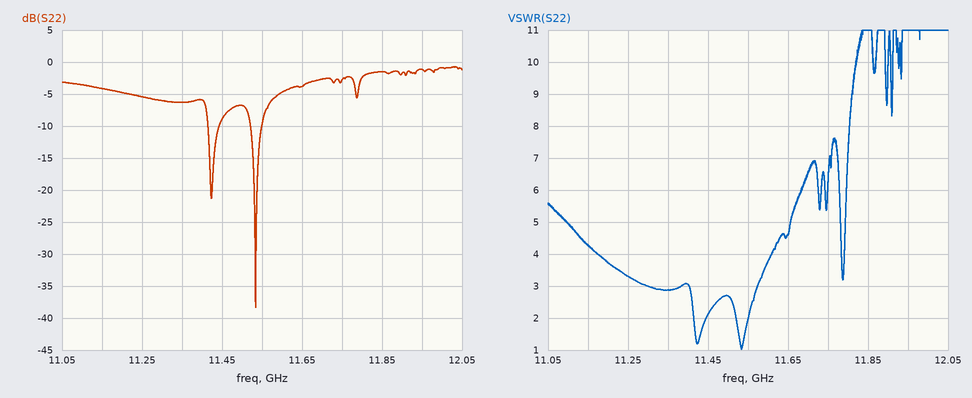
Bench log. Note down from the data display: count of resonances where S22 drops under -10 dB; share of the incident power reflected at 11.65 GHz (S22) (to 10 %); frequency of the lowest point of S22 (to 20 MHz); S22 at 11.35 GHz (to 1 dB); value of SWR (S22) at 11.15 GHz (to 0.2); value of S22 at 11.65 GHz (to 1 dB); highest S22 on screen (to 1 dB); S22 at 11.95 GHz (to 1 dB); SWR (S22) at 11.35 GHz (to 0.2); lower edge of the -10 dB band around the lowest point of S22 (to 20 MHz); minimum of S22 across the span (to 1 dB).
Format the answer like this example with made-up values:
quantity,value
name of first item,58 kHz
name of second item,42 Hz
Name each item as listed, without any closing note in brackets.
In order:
quantity,value
count of resonances where S22 drops under -10 dB,2
share of the incident power reflected at 11.65 GHz (S22),40 %
frequency of the lowest point of S22,11.54 GHz
S22 at 11.35 GHz,-6 dB
value of SWR (S22) at 11.15 GHz,4.2
value of S22 at 11.65 GHz,-4 dB
highest S22 on screen,-1 dB
S22 at 11.95 GHz,-1 dB
SWR (S22) at 11.35 GHz,2.8
lower edge of the -10 dB band around the lowest point of S22,11.52 GHz
minimum of S22 across the span,-38 dB
